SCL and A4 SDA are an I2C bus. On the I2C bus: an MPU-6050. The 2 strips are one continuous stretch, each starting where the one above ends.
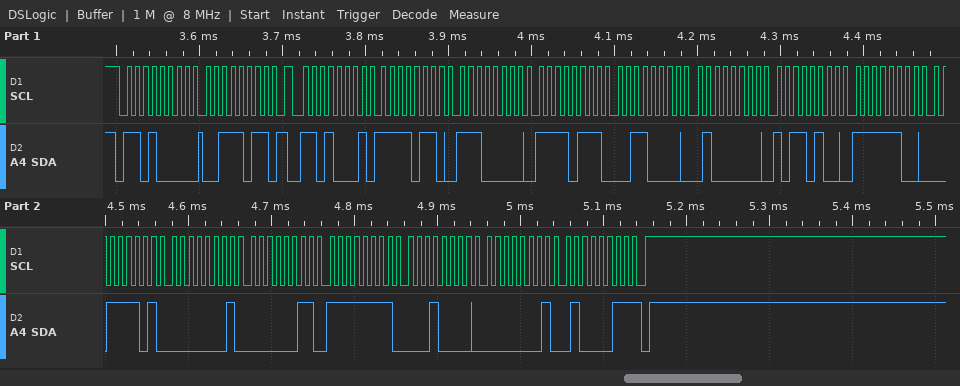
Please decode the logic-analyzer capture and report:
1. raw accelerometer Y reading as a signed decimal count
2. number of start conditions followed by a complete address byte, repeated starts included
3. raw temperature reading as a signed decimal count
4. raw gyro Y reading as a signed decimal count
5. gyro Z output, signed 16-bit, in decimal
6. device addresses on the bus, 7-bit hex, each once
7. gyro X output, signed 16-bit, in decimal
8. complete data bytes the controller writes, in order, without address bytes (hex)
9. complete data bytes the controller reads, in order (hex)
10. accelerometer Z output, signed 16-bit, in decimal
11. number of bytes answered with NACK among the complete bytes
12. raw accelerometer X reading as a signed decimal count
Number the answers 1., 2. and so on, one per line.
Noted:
1. -2256
2. 2
3. -963
4. -240
5. 323
6. 0x68
7. 259
8. 3B
9. F6 E0 F7 30 40 B4 FC 3D 01 03 FF 10 01 43
10. 16564
11. 1
12. -2336
